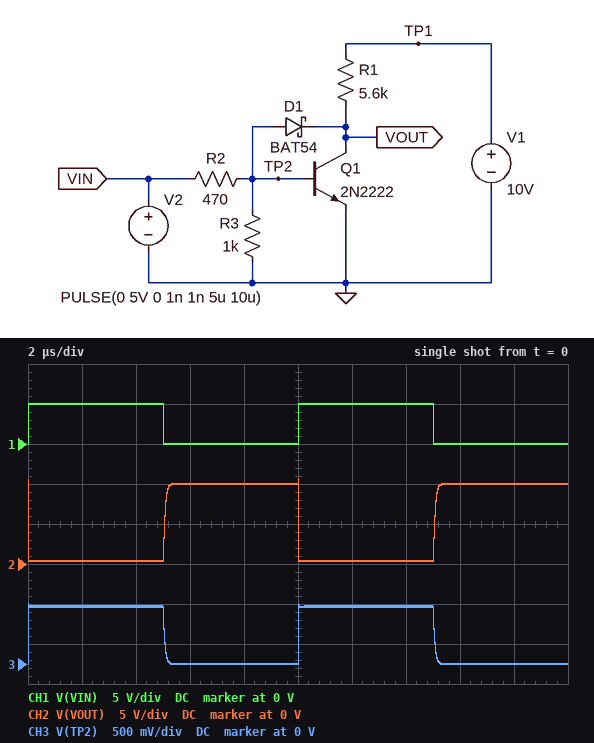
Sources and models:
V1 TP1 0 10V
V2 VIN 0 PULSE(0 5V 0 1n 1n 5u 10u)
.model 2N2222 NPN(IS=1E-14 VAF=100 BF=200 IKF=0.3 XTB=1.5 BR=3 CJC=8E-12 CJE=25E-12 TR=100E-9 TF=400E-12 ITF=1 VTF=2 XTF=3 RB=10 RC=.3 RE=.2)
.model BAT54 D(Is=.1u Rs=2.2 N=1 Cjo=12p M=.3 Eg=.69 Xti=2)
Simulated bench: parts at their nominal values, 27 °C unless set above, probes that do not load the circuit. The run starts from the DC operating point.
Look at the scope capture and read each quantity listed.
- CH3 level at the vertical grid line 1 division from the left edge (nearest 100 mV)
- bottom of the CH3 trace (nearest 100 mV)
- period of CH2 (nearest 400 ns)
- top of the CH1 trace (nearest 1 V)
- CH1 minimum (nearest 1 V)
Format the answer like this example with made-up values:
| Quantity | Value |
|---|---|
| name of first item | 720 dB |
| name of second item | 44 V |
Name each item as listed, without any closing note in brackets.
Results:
| Quantity | Value |
|---|---|
| CH3 level at the vertical grid line 1 division from the left edge | 700 mV |
| bottom of the CH3 trace | 0 V |
| period of CH2 | 10.0 µs |
| top of the CH1 trace | 5 V |
| CH1 minimum | 0 V |
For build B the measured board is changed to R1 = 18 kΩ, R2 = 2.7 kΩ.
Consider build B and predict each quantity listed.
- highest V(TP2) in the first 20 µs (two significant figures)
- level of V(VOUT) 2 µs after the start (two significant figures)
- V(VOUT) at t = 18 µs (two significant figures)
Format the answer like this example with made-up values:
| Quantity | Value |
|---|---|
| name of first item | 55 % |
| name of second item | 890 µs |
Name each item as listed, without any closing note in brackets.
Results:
| Quantity | Value |
|---|---|
| highest V(TP2) in the first 20 µs | 670 mV |
| level of V(VOUT) 2 µs after the start | 430 mV |
| V(VOUT) at t = 18 µs | 10 V |
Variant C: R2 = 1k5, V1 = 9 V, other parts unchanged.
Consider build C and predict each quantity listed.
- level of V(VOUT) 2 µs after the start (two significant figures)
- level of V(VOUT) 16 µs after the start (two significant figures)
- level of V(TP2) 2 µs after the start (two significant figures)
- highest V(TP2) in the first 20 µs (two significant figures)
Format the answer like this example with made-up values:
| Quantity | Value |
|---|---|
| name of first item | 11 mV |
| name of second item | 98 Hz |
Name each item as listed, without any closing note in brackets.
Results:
| Quantity | Value |
|---|---|
| level of V(VOUT) 2 µs after the start | 430 mV |
| level of V(VOUT) 16 µs after the start | 9.0 V |
| level of V(TP2) 2 µs after the start | 690 mV |
| highest V(TP2) in the first 20 µs | 700 mV |
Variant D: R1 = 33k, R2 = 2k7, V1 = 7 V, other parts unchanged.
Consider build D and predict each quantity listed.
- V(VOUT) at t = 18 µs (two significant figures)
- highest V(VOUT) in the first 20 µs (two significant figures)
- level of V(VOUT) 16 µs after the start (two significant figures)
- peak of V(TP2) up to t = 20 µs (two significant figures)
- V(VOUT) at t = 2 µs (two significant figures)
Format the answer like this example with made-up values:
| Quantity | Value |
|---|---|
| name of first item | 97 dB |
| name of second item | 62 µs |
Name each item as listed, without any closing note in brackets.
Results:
| Quantity | Value |
|---|---|
| V(VOUT) at t = 18 µs | 7.0 V |
| highest V(VOUT) in the first 20 µs | 7.6 V |
| level of V(VOUT) 16 µs after the start | 6.4 V |
| peak of V(TP2) up to t = 20 µs | 660 mV |
| V(VOUT) at t = 2 µs | 420 mV |
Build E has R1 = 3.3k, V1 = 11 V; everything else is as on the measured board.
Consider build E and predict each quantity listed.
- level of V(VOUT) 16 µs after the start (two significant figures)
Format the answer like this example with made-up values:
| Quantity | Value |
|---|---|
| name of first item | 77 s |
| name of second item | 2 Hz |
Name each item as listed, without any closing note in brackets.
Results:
| Quantity | Value |
|---|---|
| level of V(VOUT) 16 µs after the start | 11 V |
